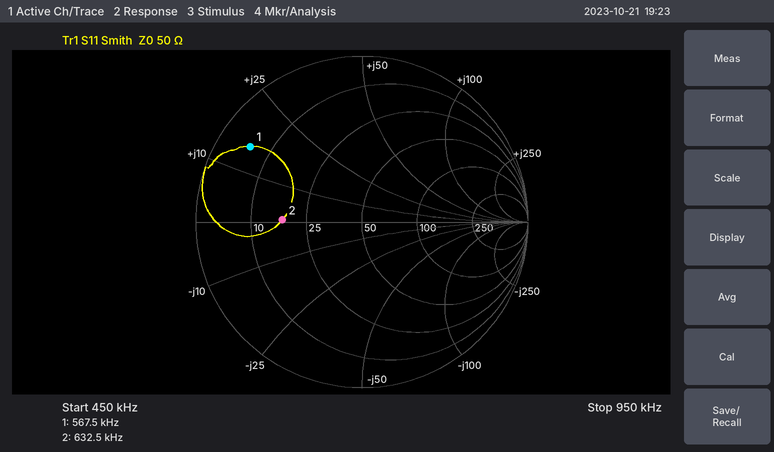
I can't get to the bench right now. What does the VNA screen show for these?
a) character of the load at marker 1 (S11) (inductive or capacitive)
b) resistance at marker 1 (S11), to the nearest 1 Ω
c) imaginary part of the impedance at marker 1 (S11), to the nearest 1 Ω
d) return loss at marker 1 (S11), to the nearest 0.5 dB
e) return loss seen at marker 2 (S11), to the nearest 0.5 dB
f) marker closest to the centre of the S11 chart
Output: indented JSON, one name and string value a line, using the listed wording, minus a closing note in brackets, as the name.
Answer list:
{
  "character of the load at marker 1 (S11)": "inductive",
  "resistance at marker 1 (S11), to the nearest 1 Ω": "6 Ω",
  "imaginary part of the impedance at marker 1 (S11), to the nearest 1 Ω": "+15 Ω",
  "return loss at marker 1 (S11), to the nearest 0.5 dB": "2.0 dB",
  "return loss seen at marker 2 (S11), to the nearest 0.5 dB": "6.5 dB",
  "marker closest to the centre of the S11 chart": "marker 2"
}
